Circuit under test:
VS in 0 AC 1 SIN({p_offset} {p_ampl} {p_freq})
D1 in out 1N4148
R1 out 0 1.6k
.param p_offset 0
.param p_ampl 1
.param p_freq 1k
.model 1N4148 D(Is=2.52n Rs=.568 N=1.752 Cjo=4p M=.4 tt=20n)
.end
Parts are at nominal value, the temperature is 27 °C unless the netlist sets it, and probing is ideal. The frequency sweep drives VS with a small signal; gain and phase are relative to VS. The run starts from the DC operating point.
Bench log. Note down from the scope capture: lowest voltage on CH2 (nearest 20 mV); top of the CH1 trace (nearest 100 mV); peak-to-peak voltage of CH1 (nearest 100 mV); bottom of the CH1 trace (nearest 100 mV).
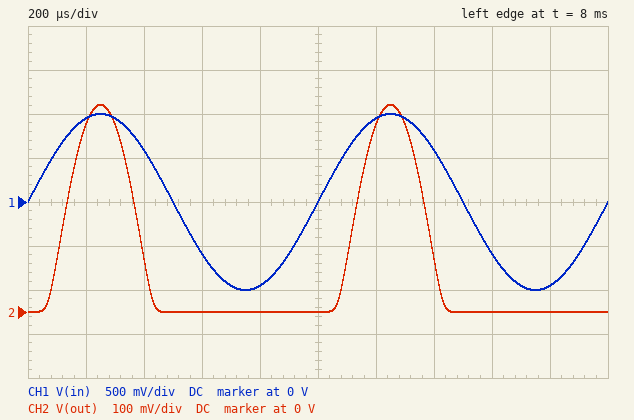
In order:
0 V
1.0 V
2.0 V
-1.0 V
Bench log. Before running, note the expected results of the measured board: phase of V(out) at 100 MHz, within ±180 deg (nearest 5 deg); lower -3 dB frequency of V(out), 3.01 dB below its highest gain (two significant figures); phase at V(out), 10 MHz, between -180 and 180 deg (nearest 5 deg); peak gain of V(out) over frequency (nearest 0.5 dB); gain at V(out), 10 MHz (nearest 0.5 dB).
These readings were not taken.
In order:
15 deg
25 MHz
70 deg
0 dB
-8.5 dB
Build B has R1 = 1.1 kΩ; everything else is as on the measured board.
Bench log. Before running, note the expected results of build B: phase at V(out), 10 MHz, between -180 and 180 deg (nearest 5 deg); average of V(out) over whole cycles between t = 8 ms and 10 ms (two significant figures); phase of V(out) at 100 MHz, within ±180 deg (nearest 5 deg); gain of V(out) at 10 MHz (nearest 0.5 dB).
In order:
75 deg
100 mV
20 deg
-11.5 dB
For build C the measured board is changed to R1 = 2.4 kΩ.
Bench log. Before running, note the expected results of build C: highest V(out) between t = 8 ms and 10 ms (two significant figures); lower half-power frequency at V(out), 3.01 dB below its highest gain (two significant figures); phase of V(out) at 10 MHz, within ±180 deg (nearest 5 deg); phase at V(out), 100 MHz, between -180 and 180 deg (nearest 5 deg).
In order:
490 mV
17 MHz
60 deg
10 deg
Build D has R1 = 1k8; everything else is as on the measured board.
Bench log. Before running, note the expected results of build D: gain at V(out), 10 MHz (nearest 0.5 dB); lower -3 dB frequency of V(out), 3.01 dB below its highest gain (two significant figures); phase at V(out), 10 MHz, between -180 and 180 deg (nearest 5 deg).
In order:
-7.5 dB
22 MHz
65 deg
